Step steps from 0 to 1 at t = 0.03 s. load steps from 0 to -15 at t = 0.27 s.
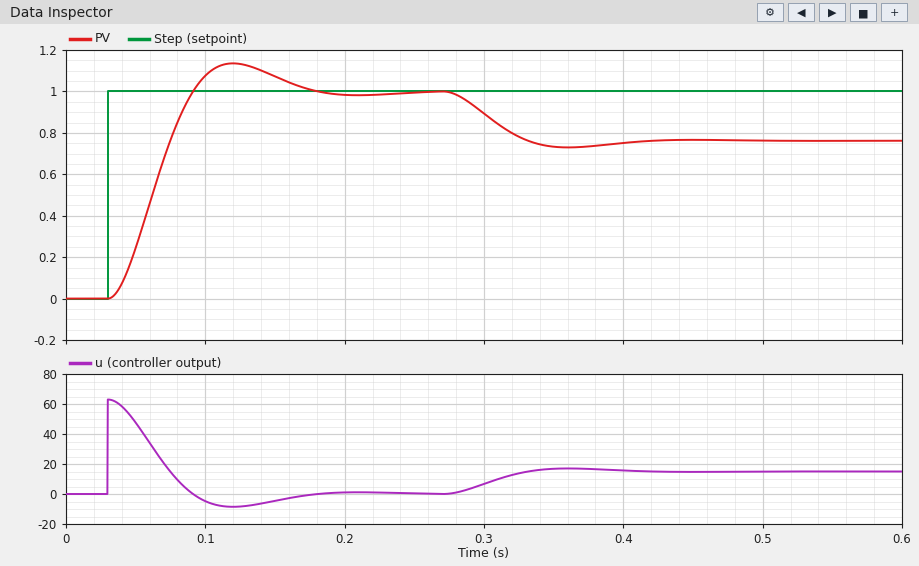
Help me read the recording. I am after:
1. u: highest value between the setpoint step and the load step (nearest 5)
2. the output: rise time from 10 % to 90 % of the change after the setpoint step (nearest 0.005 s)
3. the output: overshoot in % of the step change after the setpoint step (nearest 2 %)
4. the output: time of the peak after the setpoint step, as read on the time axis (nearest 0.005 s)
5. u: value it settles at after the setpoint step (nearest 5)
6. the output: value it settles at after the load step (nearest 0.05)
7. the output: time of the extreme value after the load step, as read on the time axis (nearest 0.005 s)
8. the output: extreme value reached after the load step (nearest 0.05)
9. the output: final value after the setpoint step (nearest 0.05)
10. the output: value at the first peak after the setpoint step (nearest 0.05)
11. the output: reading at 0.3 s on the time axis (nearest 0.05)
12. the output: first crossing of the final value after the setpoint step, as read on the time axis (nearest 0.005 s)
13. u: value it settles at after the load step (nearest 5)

65
0.040 s
14 %
0.120 s
0
0.75
0.360 s
0.75
1.00
1.15
0.90
0.090 s
15
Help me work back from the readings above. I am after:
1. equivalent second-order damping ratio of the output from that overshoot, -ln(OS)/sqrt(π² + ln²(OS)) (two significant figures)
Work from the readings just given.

0.53
